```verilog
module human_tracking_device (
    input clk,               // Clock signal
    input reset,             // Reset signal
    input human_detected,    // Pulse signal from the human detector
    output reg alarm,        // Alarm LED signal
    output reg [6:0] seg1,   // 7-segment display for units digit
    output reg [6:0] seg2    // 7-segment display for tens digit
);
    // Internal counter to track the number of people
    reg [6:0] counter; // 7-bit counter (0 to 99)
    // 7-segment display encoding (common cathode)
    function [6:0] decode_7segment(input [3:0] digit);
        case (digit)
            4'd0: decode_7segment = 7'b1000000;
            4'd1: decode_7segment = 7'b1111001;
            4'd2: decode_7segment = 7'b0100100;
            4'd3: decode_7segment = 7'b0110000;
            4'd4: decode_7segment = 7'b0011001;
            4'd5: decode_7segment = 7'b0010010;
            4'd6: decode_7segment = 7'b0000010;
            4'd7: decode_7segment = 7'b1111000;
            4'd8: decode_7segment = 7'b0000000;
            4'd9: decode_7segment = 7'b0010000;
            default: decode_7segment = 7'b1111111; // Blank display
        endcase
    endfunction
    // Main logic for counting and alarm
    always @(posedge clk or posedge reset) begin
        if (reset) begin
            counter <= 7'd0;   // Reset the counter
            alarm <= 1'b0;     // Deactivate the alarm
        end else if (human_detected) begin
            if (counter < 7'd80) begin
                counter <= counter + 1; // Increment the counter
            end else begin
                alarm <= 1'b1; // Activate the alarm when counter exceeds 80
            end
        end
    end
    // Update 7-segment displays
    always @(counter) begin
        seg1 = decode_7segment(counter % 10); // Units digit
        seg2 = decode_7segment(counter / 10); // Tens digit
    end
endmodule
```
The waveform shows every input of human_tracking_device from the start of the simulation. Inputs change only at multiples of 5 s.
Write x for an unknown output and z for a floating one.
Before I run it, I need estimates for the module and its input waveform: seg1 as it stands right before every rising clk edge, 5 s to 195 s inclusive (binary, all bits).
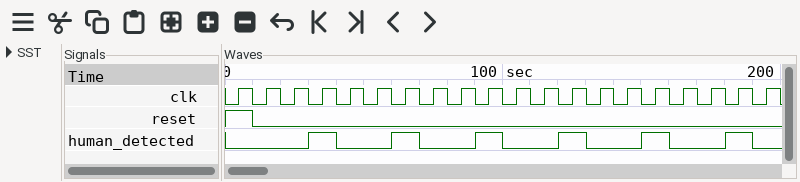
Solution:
1000000, 1000000, 1000000, 1000000, 1111001, 1111001, 1111001, 0100100, 0100100, 0100100, 0110000, 0110000, 0110000, 0011001, 0011001, 0011001, 0010010, 0010010, 0010010, 0000010
